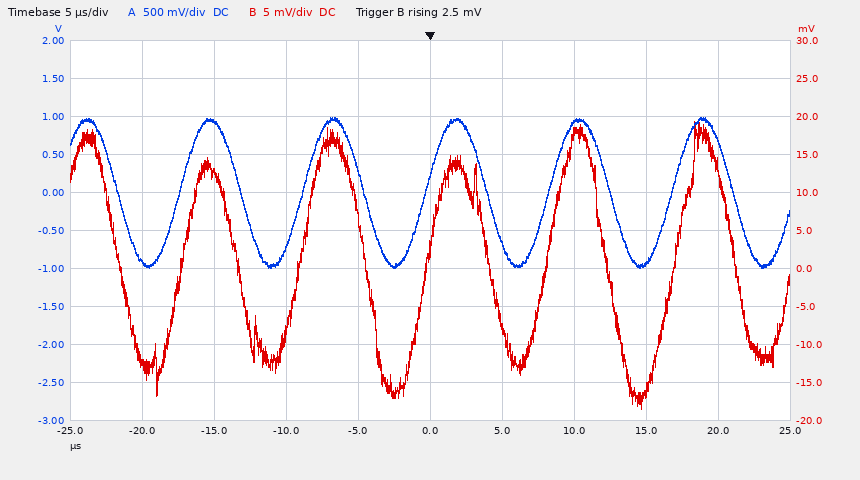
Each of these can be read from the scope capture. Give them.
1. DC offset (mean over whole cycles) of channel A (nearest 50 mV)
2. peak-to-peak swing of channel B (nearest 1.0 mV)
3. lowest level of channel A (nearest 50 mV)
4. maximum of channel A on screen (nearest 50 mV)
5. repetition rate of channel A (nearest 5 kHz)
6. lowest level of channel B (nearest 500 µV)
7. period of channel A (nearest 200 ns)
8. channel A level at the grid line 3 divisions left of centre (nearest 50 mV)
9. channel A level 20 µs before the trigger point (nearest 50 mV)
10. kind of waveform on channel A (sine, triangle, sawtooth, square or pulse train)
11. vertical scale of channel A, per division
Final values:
0 mV
38.0 mV
-1.00 V
1.00 V
115 kHz
-18.5 mV
8.6 µs
950 mV
-900 mV
sine
500 mV
